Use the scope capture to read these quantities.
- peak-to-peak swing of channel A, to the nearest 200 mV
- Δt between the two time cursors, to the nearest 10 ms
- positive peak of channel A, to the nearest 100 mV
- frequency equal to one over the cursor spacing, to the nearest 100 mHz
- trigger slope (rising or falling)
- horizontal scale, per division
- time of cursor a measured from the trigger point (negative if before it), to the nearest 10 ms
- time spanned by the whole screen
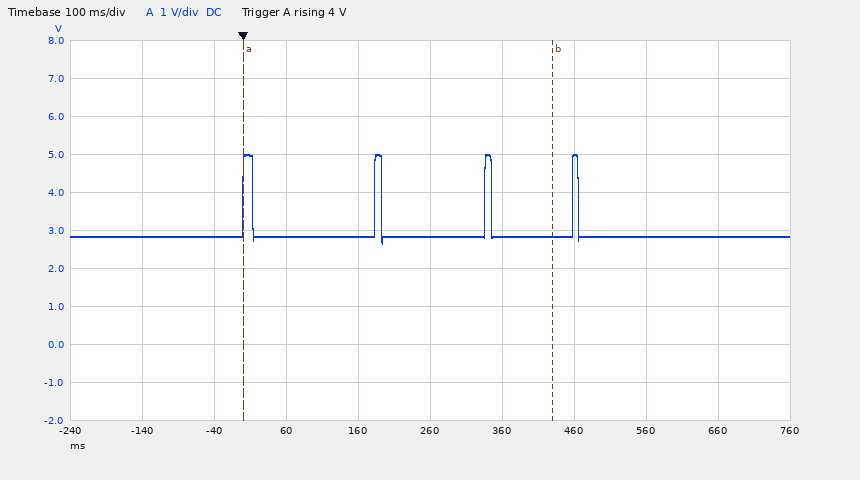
2.4 V
430 ms
5.0 V
2.3 Hz
rising
100 ms
0 ms
1 s
